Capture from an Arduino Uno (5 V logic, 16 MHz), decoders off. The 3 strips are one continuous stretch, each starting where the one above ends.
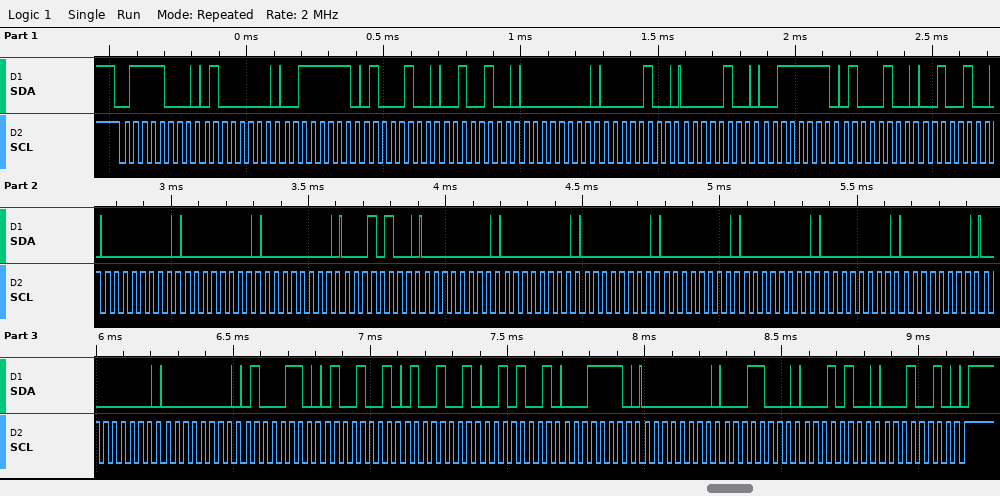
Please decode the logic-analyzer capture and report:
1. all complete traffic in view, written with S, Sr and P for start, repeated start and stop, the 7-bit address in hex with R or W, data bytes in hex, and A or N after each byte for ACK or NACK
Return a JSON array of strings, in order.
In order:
["S 3CW A 40 A 3F A 44 A 24 A 00 A 04 A 04 A 3F A 44 A 24 A 00 A 00 A 00 A 14 A 00 A 00 A 00 A 00 A 00 A 00 A 00 A 00 A 00 A 46 A 49 A 49 A 29 A 1E A 00 A 18 A 14 A 12 A P"]
